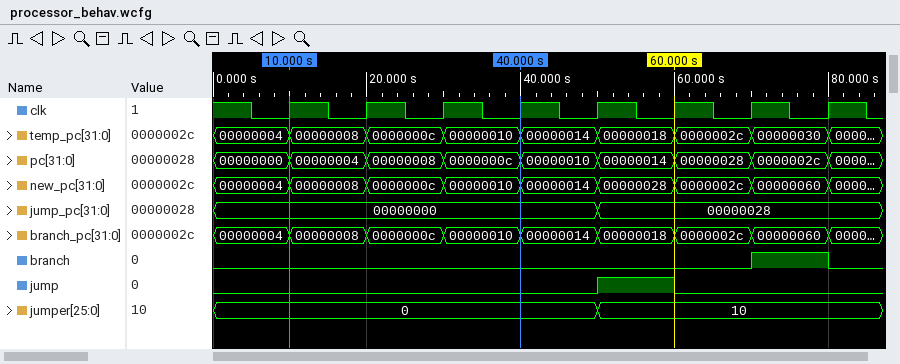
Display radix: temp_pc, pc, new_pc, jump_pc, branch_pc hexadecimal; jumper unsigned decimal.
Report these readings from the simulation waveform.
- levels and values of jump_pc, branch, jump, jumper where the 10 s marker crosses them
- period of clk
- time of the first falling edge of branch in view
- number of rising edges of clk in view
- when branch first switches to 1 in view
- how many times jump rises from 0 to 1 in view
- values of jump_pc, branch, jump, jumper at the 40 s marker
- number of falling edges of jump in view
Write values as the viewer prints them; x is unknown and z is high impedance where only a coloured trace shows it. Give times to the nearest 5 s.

jump_pc=00000000, branch=0, jump=0, jumper=0
10 s
80 s
8
70 s
1
jump_pc=00000000, branch=0, jump=0, jumper=0
1
